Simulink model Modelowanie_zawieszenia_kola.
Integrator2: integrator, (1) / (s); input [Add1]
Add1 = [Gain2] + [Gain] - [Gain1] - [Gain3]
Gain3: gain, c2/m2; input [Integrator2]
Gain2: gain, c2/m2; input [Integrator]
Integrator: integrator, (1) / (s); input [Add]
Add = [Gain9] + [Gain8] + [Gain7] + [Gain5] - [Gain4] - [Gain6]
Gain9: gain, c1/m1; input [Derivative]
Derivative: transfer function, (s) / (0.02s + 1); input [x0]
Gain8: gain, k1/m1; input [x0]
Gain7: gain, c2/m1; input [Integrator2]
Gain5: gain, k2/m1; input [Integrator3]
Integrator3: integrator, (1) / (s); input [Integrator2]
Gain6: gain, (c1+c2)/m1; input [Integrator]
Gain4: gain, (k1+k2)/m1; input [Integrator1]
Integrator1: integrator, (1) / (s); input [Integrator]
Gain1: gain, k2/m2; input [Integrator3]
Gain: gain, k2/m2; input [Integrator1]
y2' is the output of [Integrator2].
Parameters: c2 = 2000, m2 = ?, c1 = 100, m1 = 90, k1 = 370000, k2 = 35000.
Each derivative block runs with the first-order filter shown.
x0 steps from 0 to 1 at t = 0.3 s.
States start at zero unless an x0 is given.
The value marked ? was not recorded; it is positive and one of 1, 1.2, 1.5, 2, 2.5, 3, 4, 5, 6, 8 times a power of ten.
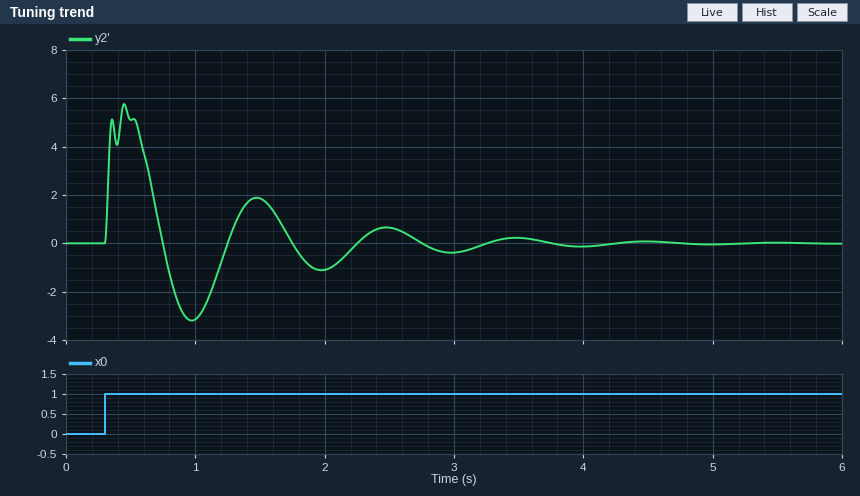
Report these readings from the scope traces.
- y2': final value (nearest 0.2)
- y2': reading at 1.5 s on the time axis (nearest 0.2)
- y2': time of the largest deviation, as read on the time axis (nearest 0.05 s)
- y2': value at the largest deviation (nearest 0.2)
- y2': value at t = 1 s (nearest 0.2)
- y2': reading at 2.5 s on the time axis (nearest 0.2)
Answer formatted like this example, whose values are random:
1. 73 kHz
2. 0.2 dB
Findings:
1. 0.0
2. 1.8
3. 0.45 s
4. 5.8
5. -3.2
6. 0.6
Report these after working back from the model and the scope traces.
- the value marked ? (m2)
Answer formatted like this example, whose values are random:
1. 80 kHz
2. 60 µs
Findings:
1. 800
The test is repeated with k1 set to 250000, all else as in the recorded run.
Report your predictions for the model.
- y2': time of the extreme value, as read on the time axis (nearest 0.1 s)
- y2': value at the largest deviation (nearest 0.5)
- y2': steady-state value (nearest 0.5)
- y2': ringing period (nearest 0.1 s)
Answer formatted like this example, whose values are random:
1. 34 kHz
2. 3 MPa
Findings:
1. 0.5 s
2. 5.5
3. 0.0
4. 1.0 s
